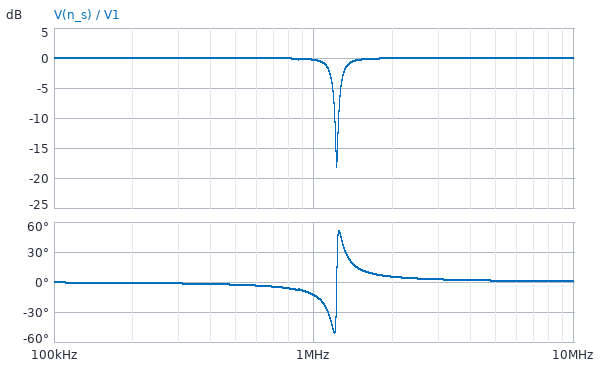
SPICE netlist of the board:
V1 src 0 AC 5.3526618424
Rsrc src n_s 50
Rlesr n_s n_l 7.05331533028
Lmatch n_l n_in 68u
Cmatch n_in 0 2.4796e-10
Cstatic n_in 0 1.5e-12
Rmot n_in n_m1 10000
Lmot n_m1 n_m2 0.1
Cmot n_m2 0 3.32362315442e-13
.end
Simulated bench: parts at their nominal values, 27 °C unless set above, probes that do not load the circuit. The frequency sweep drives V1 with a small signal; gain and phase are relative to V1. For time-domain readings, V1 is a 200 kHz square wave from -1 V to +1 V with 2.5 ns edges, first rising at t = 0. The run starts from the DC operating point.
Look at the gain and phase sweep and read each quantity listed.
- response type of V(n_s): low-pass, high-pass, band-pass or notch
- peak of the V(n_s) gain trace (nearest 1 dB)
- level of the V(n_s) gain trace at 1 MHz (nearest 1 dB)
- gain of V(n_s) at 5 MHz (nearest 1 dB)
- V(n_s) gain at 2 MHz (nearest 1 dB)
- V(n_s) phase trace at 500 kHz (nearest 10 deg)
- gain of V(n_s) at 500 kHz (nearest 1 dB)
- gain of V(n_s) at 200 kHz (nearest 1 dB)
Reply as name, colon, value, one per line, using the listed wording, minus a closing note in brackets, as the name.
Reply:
response type of V(n_s): low-pass, high-pass, band-pass or notch: notch
peak of the V(n_s) gain trace: 0 dB
level of the V(n_s) gain trace at 1 MHz: 0 dB
gain of V(n_s) at 5 MHz: 0 dB
V(n_s) gain at 2 MHz: 0 dB
V(n_s) phase trace at 500 kHz: 0 deg
gain of V(n_s) at 500 kHz: 0 dB
gain of V(n_s) at 200 kHz: 0 dB
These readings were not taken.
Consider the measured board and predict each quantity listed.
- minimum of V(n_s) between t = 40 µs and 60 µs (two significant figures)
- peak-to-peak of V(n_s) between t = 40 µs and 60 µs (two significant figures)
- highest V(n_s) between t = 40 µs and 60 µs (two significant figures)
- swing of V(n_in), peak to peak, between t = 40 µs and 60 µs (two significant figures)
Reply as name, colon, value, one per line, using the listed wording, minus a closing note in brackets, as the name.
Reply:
minimum of V(n_s) between t = 40 µs and 60 µs: -1.1 V
peak-to-peak of V(n_s) between t = 40 µs and 60 µs: 2.2 V
highest V(n_s) between t = 40 µs and 60 µs: 1.1 V
swing of V(n_in), peak to peak, between t = 40 µs and 60 µs: 4.5 V
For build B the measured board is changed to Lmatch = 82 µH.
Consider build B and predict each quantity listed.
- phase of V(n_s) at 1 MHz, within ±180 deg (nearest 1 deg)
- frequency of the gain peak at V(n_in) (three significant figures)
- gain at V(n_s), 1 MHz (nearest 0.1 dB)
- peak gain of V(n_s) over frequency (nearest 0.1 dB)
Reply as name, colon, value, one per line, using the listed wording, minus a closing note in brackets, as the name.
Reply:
phase of V(n_s) at 1 MHz, within ±180 deg: -21 deg
frequency of the gain peak at V(n_in): 1.11 MHz
gain at V(n_s), 1 MHz: -0.8 dB
peak gain of V(n_s) over frequency: 0 dB
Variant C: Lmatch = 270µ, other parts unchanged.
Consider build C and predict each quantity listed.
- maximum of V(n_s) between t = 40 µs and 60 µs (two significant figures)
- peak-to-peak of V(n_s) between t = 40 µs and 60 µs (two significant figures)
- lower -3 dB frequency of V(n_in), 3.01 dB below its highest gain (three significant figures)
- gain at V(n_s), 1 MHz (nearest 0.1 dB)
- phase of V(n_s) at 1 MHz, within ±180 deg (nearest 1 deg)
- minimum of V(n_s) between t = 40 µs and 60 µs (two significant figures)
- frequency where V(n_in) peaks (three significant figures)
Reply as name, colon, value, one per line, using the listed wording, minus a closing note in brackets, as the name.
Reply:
maximum of V(n_s) between t = 40 µs and 60 µs: 1.3 V
peak-to-peak of V(n_s) between t = 40 µs and 60 µs: 2.6 V
lower -3 dB frequency of V(n_in), 3.01 dB below its highest gain: 595 kHz
gain at V(n_s), 1 MHz: 0 dB
phase of V(n_s) at 1 MHz, within ±180 deg: 3 deg
minimum of V(n_s) between t = 40 µs and 60 µs: -1.3 V
frequency where V(n_in) peaks: 612 kHz
